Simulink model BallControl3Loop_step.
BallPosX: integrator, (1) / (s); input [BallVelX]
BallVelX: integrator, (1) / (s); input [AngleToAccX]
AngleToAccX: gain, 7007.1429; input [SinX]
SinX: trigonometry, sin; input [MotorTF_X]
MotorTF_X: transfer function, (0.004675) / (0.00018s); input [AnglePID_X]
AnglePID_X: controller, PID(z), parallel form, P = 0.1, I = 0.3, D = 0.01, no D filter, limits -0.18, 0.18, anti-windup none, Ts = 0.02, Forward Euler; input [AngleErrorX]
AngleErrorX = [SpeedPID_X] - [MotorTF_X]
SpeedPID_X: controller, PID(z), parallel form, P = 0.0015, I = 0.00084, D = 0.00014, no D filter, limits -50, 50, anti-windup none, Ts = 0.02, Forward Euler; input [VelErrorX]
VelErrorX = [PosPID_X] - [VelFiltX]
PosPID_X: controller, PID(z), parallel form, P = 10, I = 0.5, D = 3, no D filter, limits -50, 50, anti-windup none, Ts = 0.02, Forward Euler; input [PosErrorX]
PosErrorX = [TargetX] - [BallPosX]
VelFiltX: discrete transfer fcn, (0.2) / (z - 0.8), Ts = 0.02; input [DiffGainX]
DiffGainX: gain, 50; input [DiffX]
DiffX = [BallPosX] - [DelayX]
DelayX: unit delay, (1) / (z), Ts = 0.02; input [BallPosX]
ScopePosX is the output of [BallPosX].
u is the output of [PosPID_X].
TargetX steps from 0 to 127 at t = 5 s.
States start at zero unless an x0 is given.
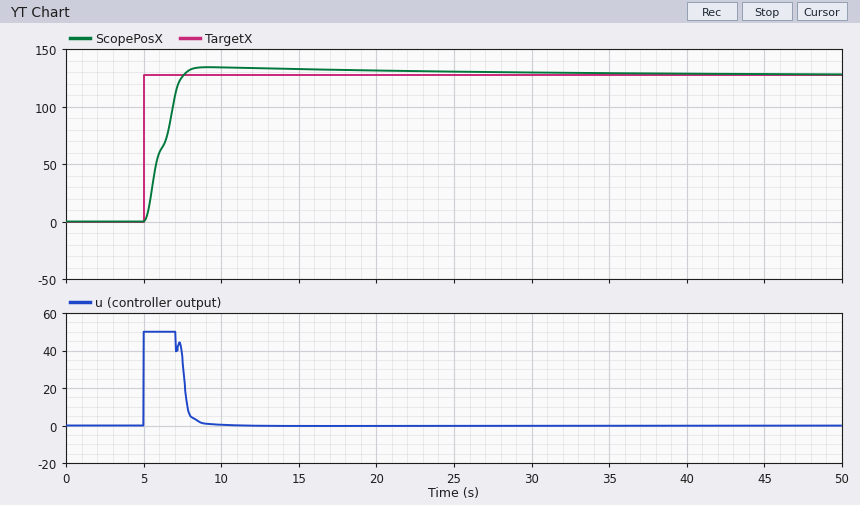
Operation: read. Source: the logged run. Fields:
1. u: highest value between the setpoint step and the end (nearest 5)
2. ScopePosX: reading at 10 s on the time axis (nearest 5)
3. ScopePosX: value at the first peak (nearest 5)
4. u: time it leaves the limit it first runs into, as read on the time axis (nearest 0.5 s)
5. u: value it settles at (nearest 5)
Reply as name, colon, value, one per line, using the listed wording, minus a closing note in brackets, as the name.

u: highest value between the setpoint step and the end: 50
ScopePosX: reading at 10 s on the time axis: 135
ScopePosX: value at the first peak: 135
u: time it leaves the limit it first runs into, as read on the time axis: 7.0 s
u: value it settles at: 0
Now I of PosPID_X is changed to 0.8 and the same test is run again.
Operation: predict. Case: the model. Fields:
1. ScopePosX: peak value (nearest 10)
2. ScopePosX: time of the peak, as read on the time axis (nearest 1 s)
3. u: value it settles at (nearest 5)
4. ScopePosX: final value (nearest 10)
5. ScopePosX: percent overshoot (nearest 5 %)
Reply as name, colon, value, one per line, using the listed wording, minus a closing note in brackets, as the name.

ScopePosX: peak value: 140
ScopePosX: time of the peak, as read on the time axis: 9 s
u: value it settles at: 0
ScopePosX: final value: 130
ScopePosX: percent overshoot: 10 %
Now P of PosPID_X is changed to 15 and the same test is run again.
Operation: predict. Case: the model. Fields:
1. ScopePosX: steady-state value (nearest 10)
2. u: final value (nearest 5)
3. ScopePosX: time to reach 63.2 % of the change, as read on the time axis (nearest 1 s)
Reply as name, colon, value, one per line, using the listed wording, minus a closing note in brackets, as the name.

ScopePosX: steady-state value: 130
u: final value: 0
ScopePosX: time to reach 63.2 % of the change, as read on the time axis: 7 s
